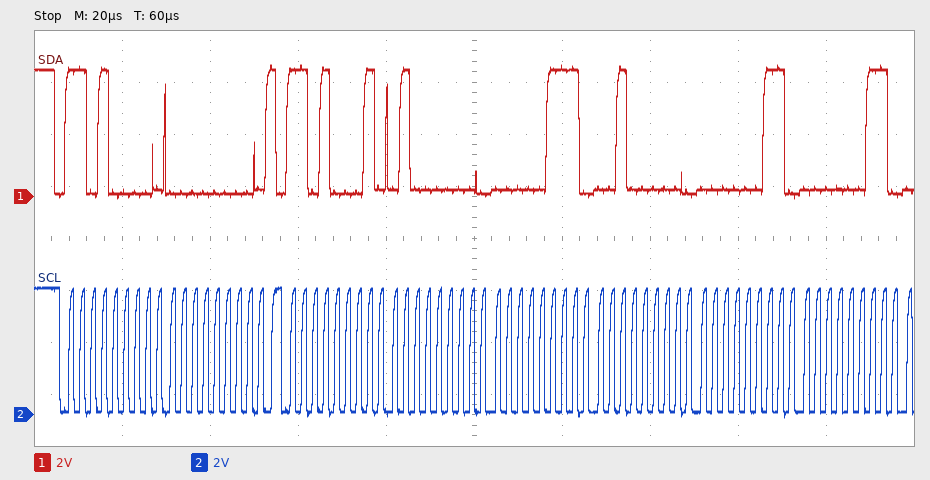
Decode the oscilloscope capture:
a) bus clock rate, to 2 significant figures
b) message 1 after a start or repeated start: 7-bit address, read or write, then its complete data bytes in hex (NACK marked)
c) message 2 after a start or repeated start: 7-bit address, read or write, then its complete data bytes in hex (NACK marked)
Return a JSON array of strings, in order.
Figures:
["400 kHz", "0x68 write: 00", "0x68 read: 40 07 20 03 03"]
